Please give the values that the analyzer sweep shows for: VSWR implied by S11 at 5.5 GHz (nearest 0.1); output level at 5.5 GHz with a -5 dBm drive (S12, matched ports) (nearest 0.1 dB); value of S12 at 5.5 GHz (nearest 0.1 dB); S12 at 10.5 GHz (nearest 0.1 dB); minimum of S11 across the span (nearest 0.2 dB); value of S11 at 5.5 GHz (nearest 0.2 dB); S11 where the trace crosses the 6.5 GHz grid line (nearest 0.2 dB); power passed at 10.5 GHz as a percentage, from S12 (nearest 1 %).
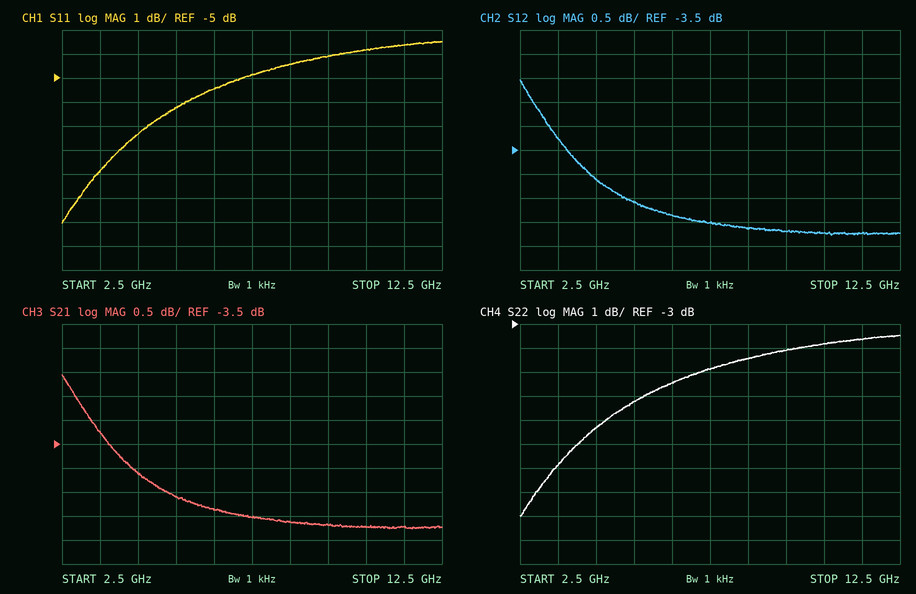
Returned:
2.9
-9.6 dBm
-4.6 dB
-5.2 dB
-11.0 dB
-6.2 dB
-5.4 dB
30 %
